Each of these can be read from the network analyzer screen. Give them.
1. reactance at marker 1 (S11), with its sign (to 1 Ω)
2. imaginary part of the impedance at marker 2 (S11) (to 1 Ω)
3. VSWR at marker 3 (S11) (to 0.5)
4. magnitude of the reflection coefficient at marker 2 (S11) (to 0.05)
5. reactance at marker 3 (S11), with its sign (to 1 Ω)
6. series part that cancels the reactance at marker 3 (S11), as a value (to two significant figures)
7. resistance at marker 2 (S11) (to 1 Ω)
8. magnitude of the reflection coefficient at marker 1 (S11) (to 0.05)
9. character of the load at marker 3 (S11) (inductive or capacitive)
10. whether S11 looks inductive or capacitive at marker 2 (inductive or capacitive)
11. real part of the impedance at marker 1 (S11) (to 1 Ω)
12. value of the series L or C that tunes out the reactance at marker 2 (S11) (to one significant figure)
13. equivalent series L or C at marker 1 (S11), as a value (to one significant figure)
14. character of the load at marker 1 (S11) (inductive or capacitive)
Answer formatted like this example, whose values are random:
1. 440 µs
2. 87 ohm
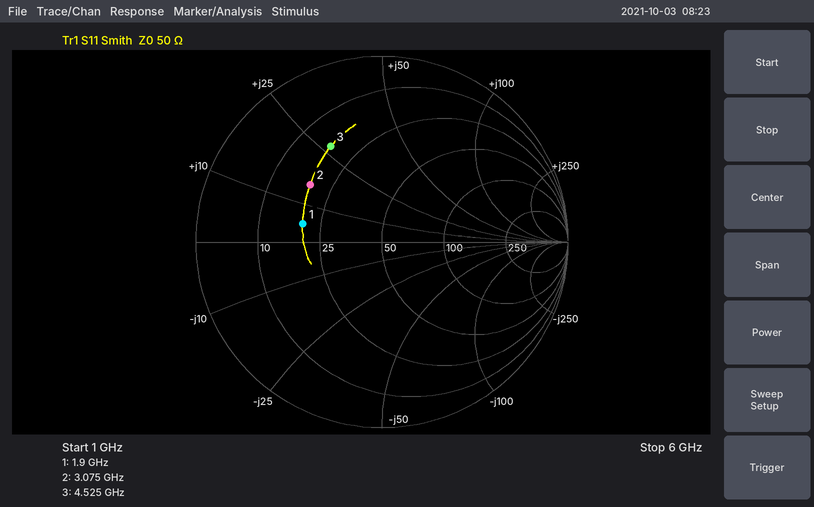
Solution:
1. +5 Ω
2. +15 Ω
3. 4.0
4. 0.50
5. +27 Ω
6. 1.3 pF
7. 19 Ω
8. 0.45
9. inductive
10. inductive
11. 20 Ω
12. 3 pF
13. 400 pH
14. inductive
